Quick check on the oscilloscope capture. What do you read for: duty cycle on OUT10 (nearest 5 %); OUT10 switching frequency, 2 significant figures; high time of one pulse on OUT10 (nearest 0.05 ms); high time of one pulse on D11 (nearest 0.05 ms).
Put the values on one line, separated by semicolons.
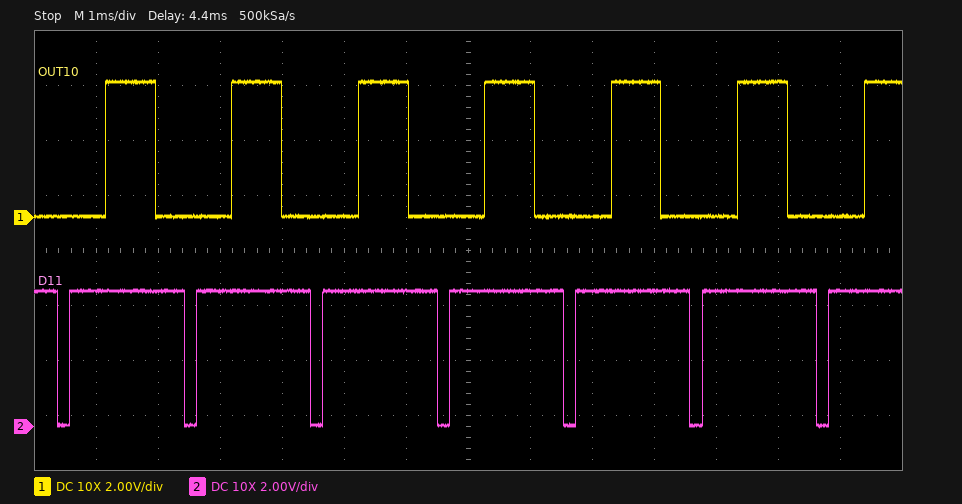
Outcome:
40 %; 490 Hz; 0.80 ms; 1.85 ms
